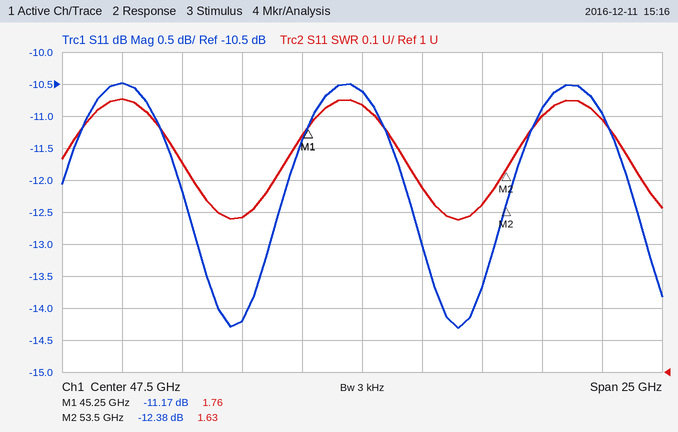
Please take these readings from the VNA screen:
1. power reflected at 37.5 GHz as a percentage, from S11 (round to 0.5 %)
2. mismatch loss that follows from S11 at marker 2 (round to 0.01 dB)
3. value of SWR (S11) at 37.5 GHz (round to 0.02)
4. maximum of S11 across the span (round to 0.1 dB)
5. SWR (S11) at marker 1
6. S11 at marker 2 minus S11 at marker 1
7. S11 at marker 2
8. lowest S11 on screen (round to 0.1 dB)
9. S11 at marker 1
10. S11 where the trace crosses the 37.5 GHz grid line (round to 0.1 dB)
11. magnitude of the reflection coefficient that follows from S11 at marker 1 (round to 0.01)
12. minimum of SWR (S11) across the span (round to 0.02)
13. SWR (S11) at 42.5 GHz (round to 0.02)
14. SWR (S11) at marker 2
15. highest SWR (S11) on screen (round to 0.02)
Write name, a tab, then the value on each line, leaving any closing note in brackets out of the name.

power reflected at 37.5 GHz as a percentage, from S11	9.0 %
mismatch loss that follows from S11 at marker 2	0.26 dB
value of SWR (S11) at 37.5 GHz	1.86
maximum of S11 across the span	-10.5 dB
SWR (S11) at marker 1	1.76
S11 at marker 2 minus S11 at marker 1	-1.21 dB
S11 at marker 2	-12.38 dB
lowest S11 on screen	-14.3 dB
S11 at marker 1	-11.17 dB
S11 where the trace crosses the 37.5 GHz grid line	-10.5 dB
magnitude of the reflection coefficient that follows from S11 at marker 1	0.28
minimum of SWR (S11) across the span	1.48
SWR (S11) at 42.5 GHz	1.48
SWR (S11) at marker 2	1.63
highest SWR (S11) on screen	1.86
